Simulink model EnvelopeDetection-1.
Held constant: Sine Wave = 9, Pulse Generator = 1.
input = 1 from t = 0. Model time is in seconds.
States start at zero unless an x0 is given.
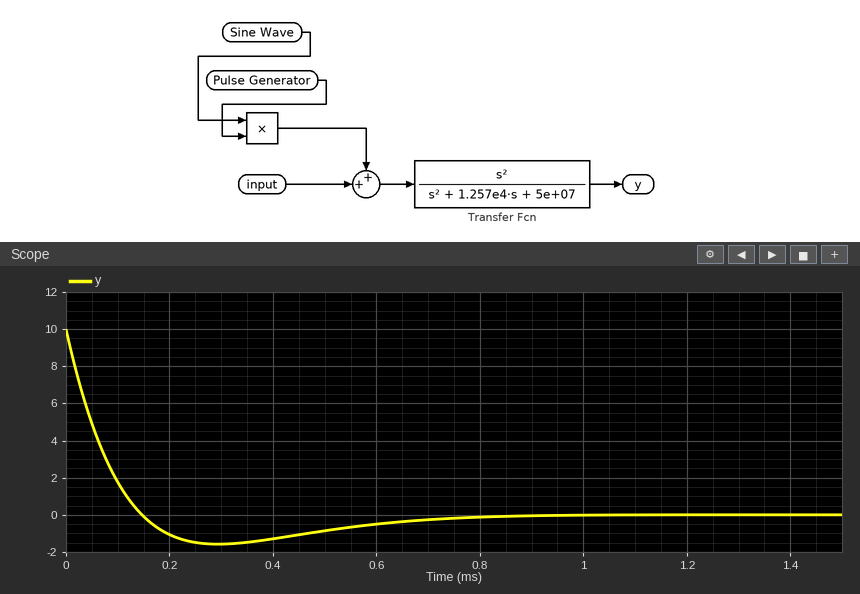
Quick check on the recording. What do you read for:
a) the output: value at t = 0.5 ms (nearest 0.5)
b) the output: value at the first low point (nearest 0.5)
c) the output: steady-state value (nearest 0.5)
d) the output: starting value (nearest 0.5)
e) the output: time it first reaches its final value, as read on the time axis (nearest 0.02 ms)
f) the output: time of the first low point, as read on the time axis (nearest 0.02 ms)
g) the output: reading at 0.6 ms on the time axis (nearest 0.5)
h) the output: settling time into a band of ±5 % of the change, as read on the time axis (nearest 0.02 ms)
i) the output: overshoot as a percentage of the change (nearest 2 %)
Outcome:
-1.0
-1.5
0.0
10.0
0.14 ms
0.30 ms
-0.5
0.60 ms
16 %
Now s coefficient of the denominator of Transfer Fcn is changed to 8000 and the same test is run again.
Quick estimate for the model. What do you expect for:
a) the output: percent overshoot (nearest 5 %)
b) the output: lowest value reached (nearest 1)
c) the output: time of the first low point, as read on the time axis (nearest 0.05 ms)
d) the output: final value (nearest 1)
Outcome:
25 %
-3
0.35 ms
0
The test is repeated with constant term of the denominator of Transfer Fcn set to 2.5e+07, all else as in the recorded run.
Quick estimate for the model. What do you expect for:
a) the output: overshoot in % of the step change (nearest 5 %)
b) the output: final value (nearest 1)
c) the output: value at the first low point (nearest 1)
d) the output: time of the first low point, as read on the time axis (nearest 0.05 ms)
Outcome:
10 %
0
-1
0.35 ms
